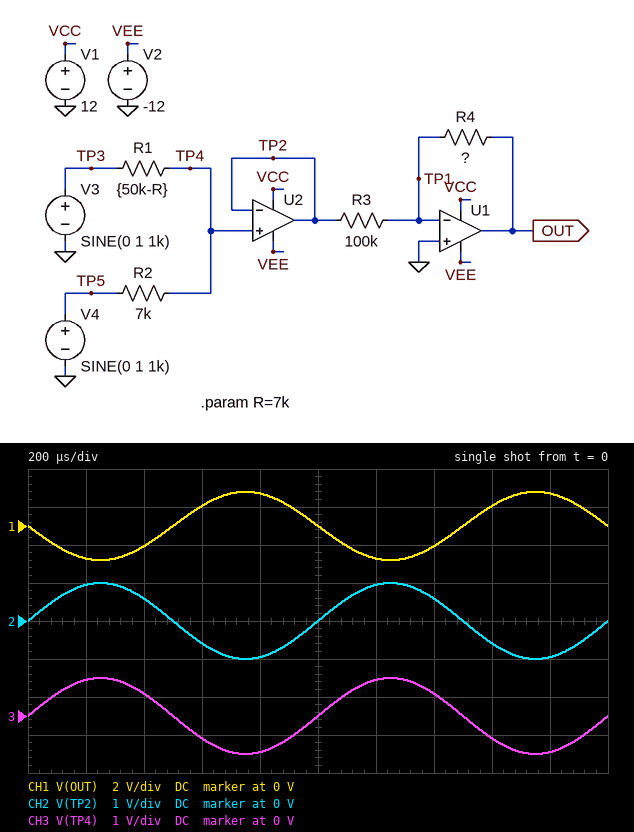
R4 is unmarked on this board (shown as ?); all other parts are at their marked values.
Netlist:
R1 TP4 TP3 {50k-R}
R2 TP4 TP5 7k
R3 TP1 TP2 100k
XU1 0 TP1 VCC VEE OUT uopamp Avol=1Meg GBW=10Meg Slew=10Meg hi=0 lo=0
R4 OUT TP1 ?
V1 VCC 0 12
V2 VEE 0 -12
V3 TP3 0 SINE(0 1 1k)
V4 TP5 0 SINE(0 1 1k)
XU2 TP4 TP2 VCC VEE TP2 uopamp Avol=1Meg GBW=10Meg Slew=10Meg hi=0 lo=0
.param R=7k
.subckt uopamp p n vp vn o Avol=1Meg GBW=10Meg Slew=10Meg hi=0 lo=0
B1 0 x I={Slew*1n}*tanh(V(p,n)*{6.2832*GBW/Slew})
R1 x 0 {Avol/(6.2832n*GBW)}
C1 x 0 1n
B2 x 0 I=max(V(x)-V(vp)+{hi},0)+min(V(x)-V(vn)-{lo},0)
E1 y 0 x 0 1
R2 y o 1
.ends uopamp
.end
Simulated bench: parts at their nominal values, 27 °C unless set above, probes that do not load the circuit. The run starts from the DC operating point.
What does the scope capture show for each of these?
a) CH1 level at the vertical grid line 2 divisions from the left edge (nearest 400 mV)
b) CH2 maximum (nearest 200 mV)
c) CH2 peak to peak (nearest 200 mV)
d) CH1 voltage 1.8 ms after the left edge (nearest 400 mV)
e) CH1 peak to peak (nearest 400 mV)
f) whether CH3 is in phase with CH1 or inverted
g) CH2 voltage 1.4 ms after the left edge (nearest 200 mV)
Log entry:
-1.2 V
1.0 V
2.0 V
1.6 V
3.6 V
inverted
600 mV
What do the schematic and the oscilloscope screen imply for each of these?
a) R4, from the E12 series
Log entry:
180 kΩ
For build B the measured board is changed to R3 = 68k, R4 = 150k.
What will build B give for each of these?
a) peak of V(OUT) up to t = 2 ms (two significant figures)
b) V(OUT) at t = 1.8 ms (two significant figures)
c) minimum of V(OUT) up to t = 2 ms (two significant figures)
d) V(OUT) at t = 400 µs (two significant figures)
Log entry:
2.2 V
2.1 V
-2.2 V
-1.3 V
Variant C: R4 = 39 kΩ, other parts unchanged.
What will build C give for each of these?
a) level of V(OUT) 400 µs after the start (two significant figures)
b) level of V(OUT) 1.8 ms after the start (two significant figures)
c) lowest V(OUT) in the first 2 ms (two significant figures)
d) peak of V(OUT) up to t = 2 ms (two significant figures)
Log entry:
-230 mV
370 mV
-390 mV
390 mV
